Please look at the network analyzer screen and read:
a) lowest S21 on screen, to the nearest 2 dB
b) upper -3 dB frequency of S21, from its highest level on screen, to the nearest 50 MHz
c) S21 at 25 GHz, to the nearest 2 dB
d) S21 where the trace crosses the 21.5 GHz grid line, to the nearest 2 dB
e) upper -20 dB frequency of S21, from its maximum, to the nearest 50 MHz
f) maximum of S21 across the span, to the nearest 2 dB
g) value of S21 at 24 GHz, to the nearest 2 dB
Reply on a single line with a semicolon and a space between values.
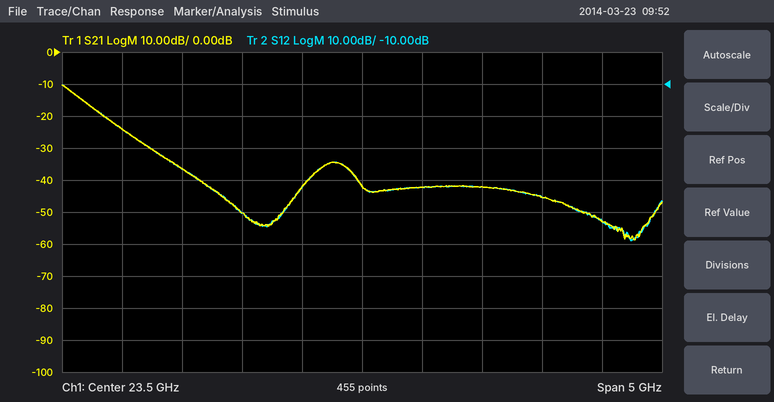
-58 dB; 21.10 GHz; -46 dB; -24 dB; 21.75 GHz; -10 dB; -42 dB
